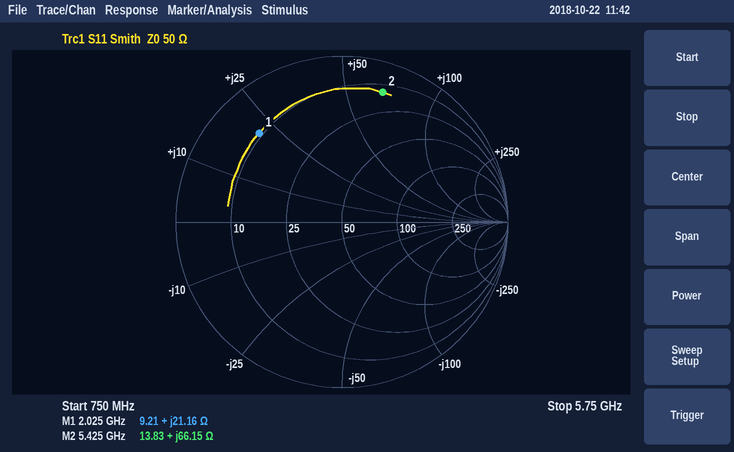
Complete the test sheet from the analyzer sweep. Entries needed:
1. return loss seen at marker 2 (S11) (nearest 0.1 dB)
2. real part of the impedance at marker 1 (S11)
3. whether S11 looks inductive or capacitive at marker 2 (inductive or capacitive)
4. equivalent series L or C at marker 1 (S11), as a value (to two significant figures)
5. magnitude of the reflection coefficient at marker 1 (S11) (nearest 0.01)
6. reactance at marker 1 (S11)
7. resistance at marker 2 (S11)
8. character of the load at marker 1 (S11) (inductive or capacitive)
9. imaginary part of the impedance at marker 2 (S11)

1.7 dB
9.21 Ω
inductive
1.7 nH
0.73
+21.16 Ω
13.83 Ω
inductive
+66.15 Ω
